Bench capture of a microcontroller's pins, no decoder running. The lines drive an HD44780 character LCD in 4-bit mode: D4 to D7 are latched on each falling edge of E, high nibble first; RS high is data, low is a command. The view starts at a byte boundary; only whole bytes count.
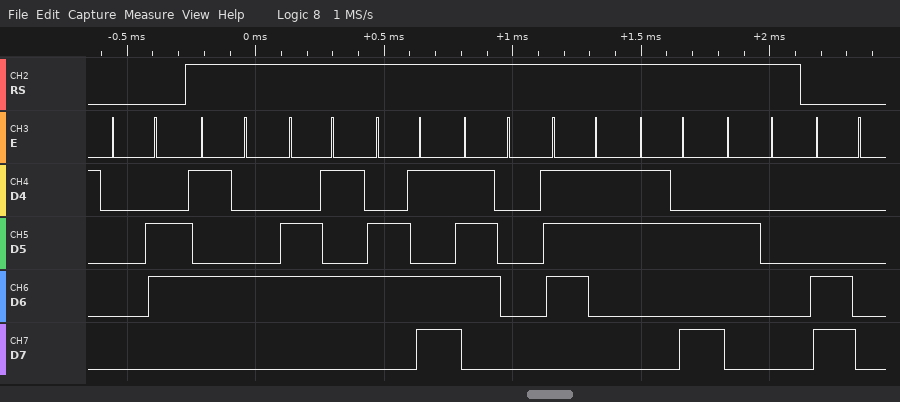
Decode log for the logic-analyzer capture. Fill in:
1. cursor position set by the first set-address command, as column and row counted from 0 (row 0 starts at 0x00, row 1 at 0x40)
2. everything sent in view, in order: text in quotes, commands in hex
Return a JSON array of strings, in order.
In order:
["column 0, row 1", "0x06 \"Temps: \" 0xC0"]
